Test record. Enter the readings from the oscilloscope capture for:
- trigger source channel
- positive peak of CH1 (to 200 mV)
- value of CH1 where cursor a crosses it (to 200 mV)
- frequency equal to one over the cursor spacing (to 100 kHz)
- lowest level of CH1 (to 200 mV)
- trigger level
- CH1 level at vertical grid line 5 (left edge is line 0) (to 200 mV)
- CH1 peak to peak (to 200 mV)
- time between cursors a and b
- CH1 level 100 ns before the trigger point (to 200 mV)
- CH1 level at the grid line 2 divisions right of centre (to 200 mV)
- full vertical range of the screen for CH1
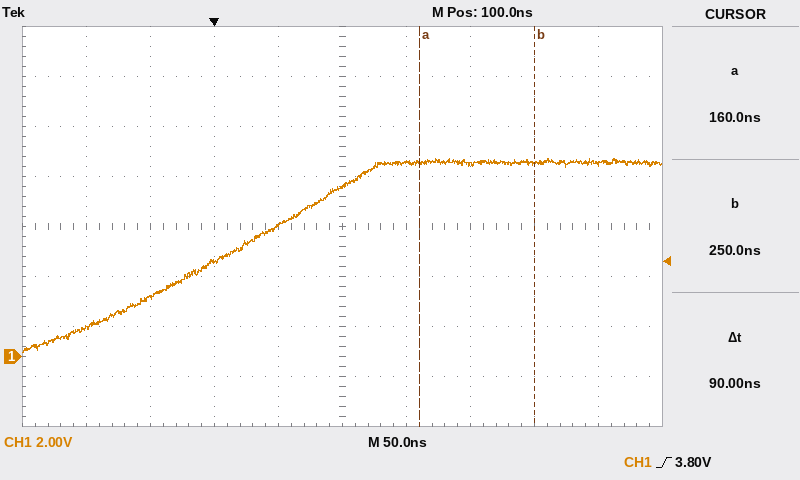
CH1
8.0 V
7.8 V
11.1 MHz
200 mV
3.80 V
6.8 V
7.8 V
90 ns
1.2 V
7.6 V
16 V
